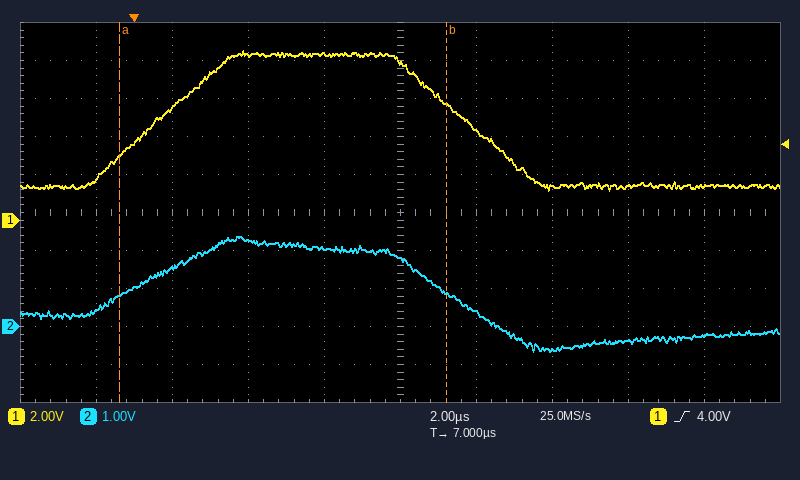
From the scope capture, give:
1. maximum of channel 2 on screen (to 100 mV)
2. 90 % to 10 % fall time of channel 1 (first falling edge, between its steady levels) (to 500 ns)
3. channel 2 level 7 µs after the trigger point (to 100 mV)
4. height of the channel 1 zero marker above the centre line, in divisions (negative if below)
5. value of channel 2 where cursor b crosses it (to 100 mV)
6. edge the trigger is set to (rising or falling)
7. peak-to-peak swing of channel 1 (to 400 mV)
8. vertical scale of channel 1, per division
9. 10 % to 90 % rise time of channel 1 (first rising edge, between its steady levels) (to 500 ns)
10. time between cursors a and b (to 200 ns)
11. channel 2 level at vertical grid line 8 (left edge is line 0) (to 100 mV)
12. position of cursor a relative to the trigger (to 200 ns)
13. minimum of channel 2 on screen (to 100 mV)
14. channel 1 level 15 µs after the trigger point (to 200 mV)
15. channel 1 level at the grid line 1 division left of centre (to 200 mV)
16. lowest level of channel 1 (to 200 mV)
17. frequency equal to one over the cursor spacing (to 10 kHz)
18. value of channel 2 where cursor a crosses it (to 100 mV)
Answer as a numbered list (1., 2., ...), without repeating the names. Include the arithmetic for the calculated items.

1. 2.4 V
2. 3.0 µs
3. 1.8 V
4. -0.2 div
5. 900 mV
6. rising
7. 7.2 V
8. 2 V
9. 3.0 µs
10. 8.6 µs
11. -400 mV
12. -400 ns
13. -700 mV
14. 1.8 V
15. 8.8 V
16. 1.6 V
17. 1 / 8.6 µs ≈ 120 kHz
18. 800 mV
